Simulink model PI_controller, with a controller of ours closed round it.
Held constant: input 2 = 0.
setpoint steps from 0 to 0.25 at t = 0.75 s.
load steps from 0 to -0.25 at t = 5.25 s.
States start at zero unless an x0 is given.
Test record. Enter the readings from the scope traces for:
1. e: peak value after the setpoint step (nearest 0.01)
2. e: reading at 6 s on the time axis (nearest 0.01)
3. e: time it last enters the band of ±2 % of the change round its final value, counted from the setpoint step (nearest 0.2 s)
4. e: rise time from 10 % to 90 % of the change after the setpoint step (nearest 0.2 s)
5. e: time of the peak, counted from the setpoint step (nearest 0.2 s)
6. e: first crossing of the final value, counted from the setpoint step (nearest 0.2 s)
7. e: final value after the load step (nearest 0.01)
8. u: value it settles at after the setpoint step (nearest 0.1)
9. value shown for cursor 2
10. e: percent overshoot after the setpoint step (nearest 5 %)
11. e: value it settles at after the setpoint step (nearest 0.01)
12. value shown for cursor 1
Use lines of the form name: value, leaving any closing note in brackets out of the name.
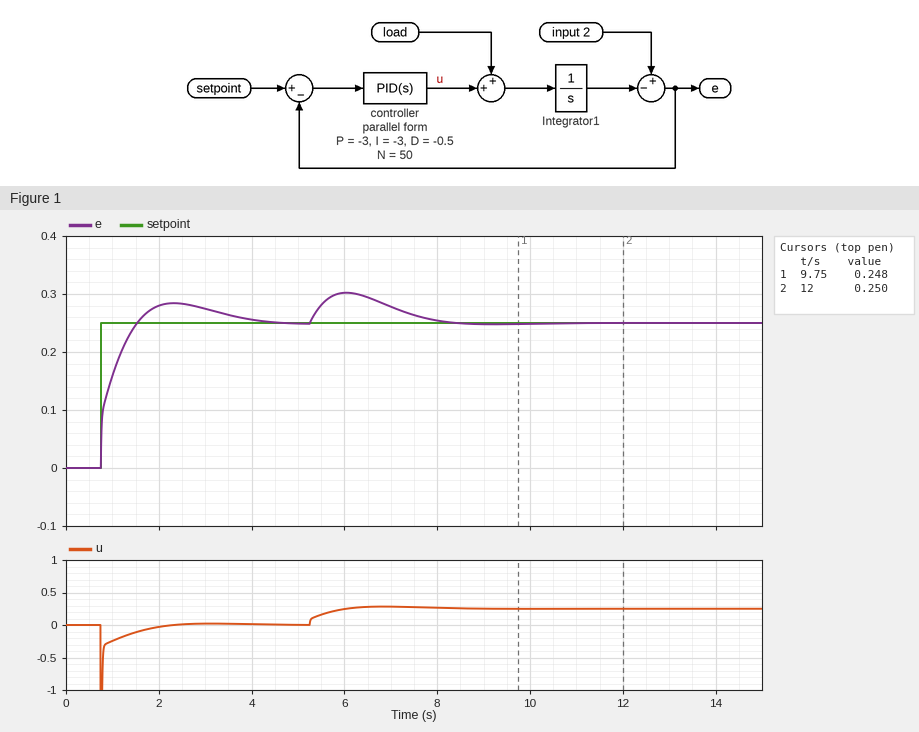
e: peak value after the setpoint step: 0.28
e: reading at 6 s on the time axis: 0.30
e: time it last enters the band of ±2 % of the change round its final value, counted from the setpoint step: 3.4 s
e: rise time from 10 % to 90 % of the change after the setpoint step: 0.6 s
e: time of the peak, counted from the setpoint step: 1.6 s
e: first crossing of the final value, counted from the setpoint step: 0.8 s
e: final value after the load step: 0.25
u: value it settles at after the setpoint step: 0.0
value shown for cursor 2: 0.250
e: percent overshoot after the setpoint step: 15 %
e: value it settles at after the setpoint step: 0.25
value shown for cursor 1: 0.248
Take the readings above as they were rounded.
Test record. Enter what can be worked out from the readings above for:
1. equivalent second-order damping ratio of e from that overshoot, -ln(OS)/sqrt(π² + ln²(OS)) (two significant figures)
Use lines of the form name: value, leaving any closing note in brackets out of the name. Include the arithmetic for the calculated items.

equivalent second-order damping ratio of e from that overshoot, -ln(OS)/sqrt(π² + ln²(OS)): ln(0.15) = -1.897; 1.897 / sqrt(9.870 + 3.599) = 0.52
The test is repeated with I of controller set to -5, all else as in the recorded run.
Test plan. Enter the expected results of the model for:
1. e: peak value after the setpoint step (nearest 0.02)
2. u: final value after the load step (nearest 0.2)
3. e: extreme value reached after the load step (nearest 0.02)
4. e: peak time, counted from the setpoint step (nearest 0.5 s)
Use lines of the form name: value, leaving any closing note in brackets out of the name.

e: peak value after the setpoint step: 0.30
u: final value after the load step: 0.2
e: extreme value reached after the load step: 0.30
e: peak time, counted from the setpoint step: 1.5 s
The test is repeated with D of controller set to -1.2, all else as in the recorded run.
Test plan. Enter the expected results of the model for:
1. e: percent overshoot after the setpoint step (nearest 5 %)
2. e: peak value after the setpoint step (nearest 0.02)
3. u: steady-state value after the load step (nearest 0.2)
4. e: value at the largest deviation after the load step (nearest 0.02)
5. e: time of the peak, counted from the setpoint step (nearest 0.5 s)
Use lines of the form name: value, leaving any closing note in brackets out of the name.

e: percent overshoot after the setpoint step: 10 %
e: peak value after the setpoint step: 0.28
u: steady-state value after the load step: 0.2
e: value at the largest deviation after the load step: 0.30
e: time of the peak, counted from the setpoint step: 2.0 s
